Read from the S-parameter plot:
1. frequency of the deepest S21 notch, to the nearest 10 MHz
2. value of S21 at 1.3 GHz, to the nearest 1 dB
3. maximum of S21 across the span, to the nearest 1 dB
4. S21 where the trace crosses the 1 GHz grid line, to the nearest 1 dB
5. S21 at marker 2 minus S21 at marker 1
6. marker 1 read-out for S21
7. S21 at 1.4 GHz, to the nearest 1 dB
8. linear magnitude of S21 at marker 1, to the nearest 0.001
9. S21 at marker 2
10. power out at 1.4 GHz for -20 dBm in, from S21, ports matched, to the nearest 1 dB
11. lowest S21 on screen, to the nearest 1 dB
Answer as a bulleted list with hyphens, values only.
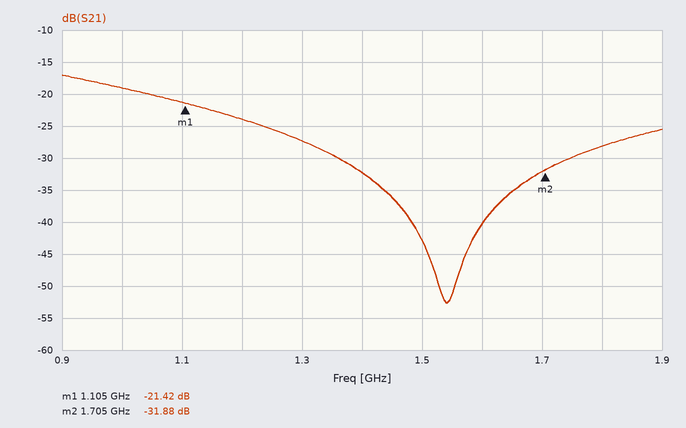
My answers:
- 1.54 GHz
- -27 dB
- -17 dB
- -19 dB
- -10.46 dB
- -21.42 dB
- -32 dB
- 0.085
- -31.88 dB
- -52 dBm
- -53 dB
